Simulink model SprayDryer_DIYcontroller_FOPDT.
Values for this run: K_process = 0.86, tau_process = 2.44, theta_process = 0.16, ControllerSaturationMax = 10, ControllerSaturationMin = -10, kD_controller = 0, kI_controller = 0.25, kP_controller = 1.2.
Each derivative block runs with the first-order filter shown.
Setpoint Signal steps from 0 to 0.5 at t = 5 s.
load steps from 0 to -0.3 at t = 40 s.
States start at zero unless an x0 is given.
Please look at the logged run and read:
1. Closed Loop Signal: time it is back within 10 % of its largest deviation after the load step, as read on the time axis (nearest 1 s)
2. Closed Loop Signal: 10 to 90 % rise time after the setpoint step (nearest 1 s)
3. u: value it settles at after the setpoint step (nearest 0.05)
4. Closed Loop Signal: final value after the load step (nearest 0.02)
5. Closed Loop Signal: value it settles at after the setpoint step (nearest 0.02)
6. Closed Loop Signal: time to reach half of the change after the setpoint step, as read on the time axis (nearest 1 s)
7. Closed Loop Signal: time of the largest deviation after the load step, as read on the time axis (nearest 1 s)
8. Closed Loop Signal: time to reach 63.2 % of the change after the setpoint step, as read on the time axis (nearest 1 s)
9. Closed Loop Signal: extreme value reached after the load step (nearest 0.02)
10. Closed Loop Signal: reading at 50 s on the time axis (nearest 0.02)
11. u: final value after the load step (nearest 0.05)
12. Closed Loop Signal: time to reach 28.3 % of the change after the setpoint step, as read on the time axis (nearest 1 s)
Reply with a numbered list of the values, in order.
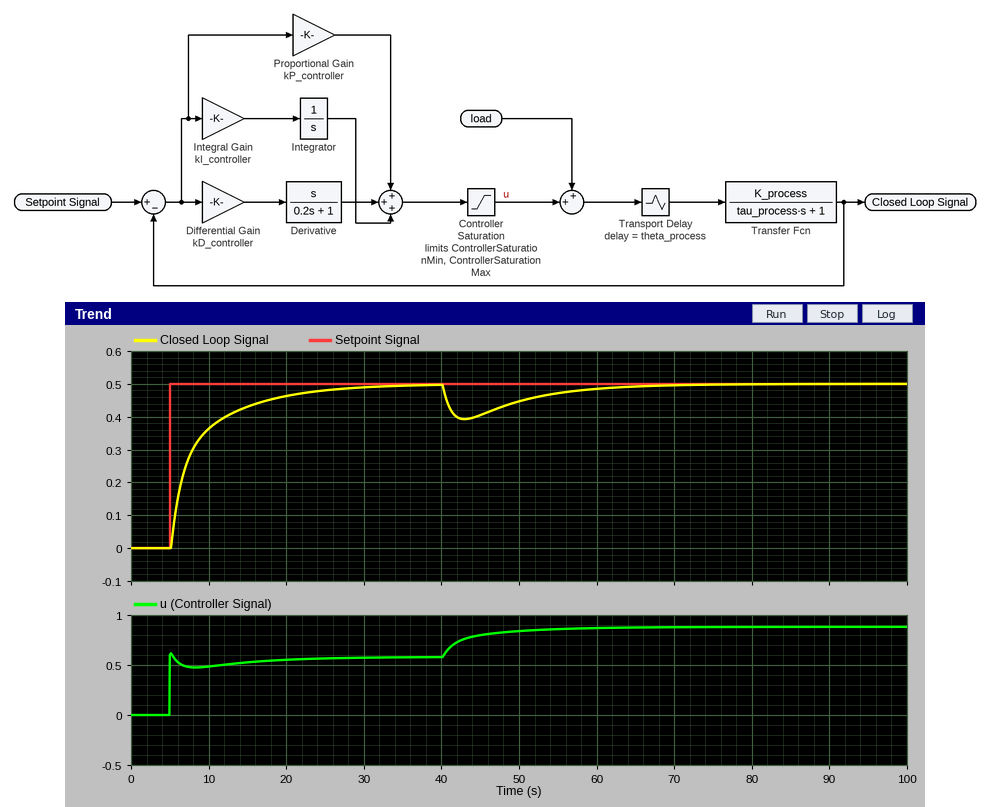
1. 63 s
2. 12 s
3. 0.60
4. 0.50
5. 0.50
6. 7 s
7. 43 s
8. 8 s
9. 0.40
10. 0.44
11. 0.90
12. 6 s
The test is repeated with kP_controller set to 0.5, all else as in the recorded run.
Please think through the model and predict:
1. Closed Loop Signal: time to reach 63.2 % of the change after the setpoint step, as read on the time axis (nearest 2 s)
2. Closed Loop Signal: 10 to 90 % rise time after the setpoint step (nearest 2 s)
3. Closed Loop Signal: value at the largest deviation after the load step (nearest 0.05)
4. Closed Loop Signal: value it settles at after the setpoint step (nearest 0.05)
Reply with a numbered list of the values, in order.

1. 10 s
2. 10 s
3. 0.35
4. 0.50
